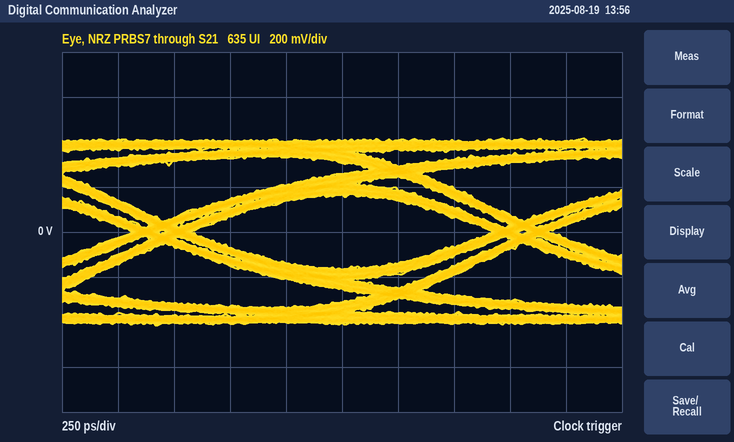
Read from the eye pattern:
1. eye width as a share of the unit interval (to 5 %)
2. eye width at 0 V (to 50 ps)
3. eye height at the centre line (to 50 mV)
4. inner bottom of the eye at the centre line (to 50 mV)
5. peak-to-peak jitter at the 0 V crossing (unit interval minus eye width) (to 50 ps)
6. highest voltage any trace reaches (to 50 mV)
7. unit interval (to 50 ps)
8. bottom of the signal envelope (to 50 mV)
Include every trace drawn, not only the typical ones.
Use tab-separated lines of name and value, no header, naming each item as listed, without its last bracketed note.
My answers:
eye width as a share of the unit interval	85 %
eye width at 0 V	1.35 ns
eye height at the centre line	350 mV
inner bottom of the eye at the centre line	-150 mV
peak-to-peak jitter at the 0 V crossing (unit interval minus eye width)	250 ps
highest voltage any trace reaches	400 mV
unit interval	1.60 ns
bottom of the signal envelope	-400 mV
